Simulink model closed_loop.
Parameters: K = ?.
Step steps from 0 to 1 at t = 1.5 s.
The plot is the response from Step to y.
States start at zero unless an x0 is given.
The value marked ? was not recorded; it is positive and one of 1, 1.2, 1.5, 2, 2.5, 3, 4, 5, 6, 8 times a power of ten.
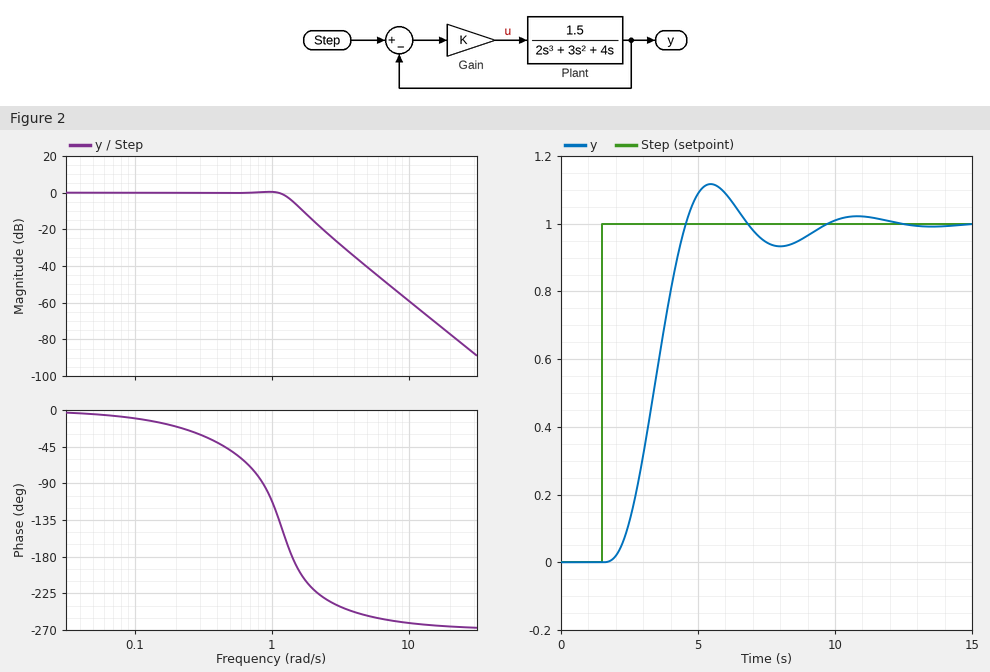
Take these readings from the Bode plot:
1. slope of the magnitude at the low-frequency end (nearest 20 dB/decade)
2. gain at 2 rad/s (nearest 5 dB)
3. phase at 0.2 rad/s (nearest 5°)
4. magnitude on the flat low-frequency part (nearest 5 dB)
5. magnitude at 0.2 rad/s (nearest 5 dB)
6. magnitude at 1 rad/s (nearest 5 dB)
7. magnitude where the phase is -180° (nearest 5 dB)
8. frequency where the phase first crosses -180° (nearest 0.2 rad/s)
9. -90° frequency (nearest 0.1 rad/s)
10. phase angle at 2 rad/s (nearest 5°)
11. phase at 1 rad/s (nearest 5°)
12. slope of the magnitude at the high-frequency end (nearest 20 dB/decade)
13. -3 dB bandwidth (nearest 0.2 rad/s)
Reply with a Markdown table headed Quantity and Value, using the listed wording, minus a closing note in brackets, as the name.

| Quantity | Value |
|---|---|
| slope of the magnitude at the low-frequency end | 0 dB/decade |
| gain at 2 rad/s | -15 dB |
| phase at 0.2 rad/s | -20° |
| magnitude on the flat low-frequency part | 0 dB |
| magnitude at 0.2 rad/s | 0 dB |
| magnitude at 1 rad/s | 0 dB |
| magnitude where the phase is -180° | -5 dB |
| frequency where the phase first crosses -180° | 1.4 rad/s |
| -90° frequency | 0.9 rad/s |
| phase angle at 2 rad/s | -220° |
| phase at 1 rad/s | -110° |
| slope of the magnitude at the high-frequency end | -60 dB/decade |
| -3 dB bandwidth | 1.4 rad/s |
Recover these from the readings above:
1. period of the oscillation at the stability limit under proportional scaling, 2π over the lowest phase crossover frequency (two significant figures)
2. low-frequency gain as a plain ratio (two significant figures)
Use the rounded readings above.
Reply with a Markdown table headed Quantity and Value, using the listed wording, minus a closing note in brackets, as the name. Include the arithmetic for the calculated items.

| Quantity | Value |
|---|---|
| period of the oscillation at the stability limit under proportional scaling, 2π over the lowest phase crossover frequency | 2π / 1.4 = 4.5 s |
| low-frequency gain as a plain ratio | 10^(0 / 20) = 1.0 |
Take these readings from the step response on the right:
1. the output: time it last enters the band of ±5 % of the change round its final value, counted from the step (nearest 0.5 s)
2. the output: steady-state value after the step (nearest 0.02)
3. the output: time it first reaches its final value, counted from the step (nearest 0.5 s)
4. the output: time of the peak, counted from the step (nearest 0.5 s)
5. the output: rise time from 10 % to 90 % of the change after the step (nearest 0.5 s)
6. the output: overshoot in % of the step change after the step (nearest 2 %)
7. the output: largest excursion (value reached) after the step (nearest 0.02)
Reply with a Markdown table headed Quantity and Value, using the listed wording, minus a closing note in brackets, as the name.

| Quantity | Value |
|---|---|
| the output: time it last enters the band of ±5 % of the change round its final value, counted from the step | 7.0 s |
| the output: steady-state value after the step | 1.00 |
| the output: time it first reaches its final value, counted from the step | 3.0 s |
| the output: time of the peak, counted from the step | 4.0 s |
| the output: rise time from 10 % to 90 % of the change after the step | 2.0 s |
| the output: overshoot in % of the step change after the step | 12 % |
| the output: largest excursion (value reached) after the step | 1.12 |
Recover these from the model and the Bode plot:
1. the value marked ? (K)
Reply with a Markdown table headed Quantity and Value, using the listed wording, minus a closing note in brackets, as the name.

| Quantity | Value |
|---|---|
| the value marked ? | 1.5 |
